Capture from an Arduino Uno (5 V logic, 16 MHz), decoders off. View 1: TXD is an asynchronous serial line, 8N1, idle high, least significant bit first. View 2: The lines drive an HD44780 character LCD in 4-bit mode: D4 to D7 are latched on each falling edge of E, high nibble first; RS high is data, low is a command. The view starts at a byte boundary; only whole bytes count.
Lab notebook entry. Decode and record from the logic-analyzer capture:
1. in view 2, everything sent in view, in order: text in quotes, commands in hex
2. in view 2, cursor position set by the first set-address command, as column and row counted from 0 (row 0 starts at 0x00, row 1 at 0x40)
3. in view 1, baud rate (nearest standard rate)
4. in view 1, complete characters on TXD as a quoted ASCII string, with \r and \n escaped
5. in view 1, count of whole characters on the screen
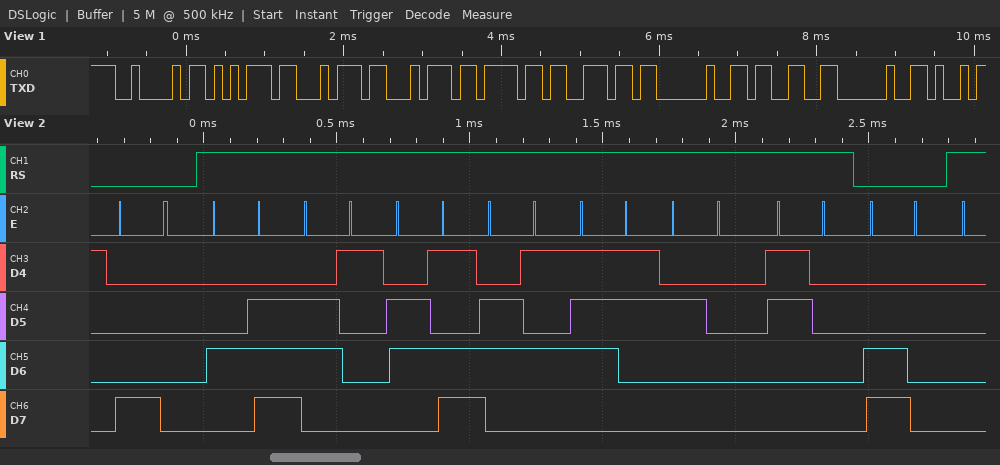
0x80 "Names 0" 0xC0
column 0, row 0
9600 baud
"Button 3 "
9
